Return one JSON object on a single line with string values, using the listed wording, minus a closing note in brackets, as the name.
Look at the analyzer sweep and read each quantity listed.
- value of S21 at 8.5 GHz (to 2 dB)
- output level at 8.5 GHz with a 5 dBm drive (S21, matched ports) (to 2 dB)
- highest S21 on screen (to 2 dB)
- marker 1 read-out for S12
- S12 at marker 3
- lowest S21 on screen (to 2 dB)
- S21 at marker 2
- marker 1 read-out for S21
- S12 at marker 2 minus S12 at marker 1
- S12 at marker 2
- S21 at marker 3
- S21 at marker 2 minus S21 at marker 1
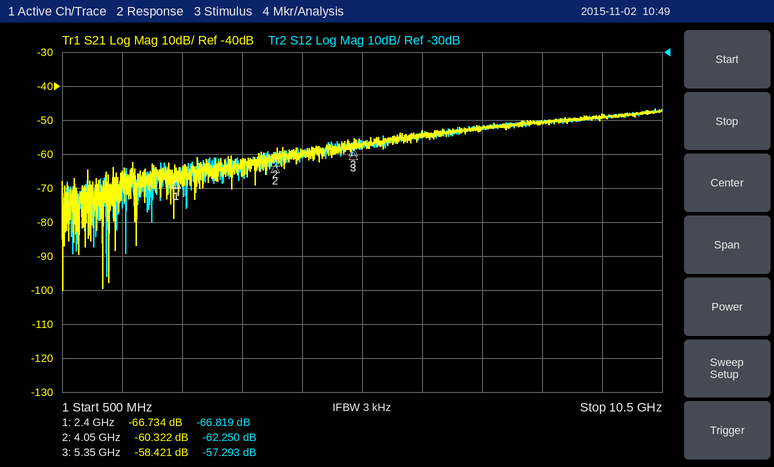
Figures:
{"value of S21 at 8.5 GHz": "-50 dB", "output level at 8.5 GHz with a 5 dBm drive (S21, matched ports)": "-46 dBm", "highest S21 on screen": "-46 dB", "marker 1 read-out for S12": "-66.819 dB", "S12 at marker 3": "-57.293 dB", "lowest S21 on screen": "-100 dB", "S21 at marker 2": "-60.322 dB", "marker 1 read-out for S21": "-66.734 dB", "S12 at marker 2 minus S12 at marker 1": "4.569 dB", "S12 at marker 2": "-62.250 dB", "S21 at marker 3": "-58.421 dB", "S21 at marker 2 minus S21 at marker 1": "6.412 dB"}
